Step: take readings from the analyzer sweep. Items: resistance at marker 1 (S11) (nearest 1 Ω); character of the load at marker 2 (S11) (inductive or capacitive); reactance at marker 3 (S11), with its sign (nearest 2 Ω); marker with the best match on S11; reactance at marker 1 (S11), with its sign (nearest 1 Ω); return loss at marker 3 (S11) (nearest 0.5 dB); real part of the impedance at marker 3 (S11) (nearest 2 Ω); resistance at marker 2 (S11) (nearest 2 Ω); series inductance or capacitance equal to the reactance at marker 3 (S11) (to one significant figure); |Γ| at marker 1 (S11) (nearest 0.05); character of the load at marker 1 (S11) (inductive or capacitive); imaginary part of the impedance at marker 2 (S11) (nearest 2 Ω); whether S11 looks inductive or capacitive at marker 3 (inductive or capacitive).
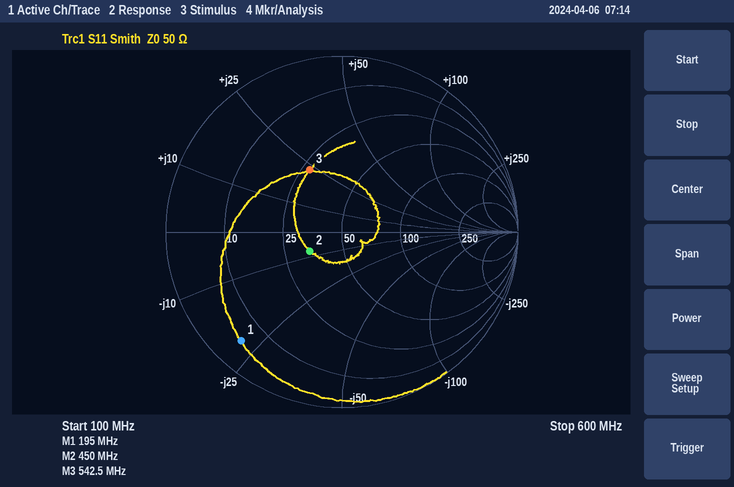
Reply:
5 Ω
capacitive
+24 Ω
marker 2
-22 Ω
8.0 dB
28 Ω
34 Ω
7 nH
0.85
capacitive
-8 Ω
inductive
